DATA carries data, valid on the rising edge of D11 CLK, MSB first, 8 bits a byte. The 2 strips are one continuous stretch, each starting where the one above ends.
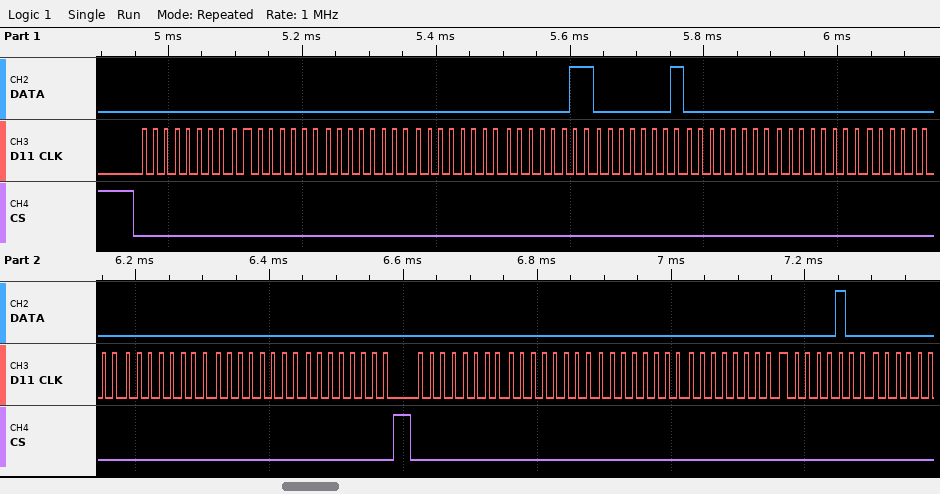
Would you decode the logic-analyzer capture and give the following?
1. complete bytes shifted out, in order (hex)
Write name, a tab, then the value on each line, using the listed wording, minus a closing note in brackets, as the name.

complete bytes shifted out, in order	00 00 00 00 03 01 00 00 00 00 00 00 00 00 00 00 04
